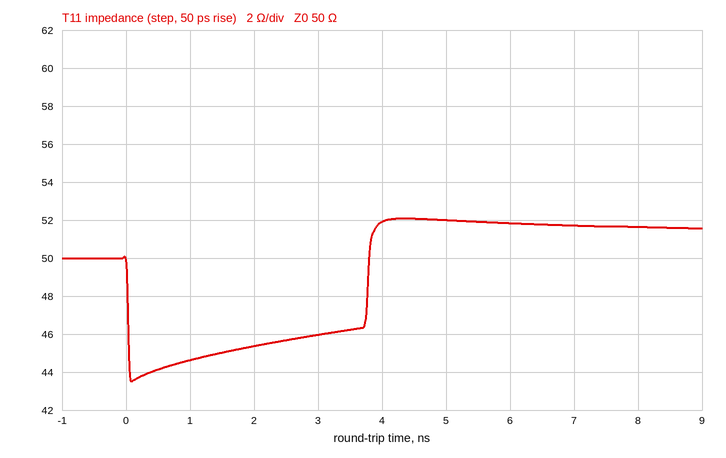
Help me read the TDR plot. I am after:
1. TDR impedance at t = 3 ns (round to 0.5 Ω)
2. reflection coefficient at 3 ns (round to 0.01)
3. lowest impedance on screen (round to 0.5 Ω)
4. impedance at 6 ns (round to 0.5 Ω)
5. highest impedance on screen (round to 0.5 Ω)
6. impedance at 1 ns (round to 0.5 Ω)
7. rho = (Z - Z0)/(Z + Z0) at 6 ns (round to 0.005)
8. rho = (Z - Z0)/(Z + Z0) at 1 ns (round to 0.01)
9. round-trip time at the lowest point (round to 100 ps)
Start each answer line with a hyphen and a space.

- 46.0 Ω
- -0.04
- 43.5 Ω
- 52.0 Ω
- 52.0 Ω
- 44.5 Ω
- +0.020
- -0.06
- 100 ps
